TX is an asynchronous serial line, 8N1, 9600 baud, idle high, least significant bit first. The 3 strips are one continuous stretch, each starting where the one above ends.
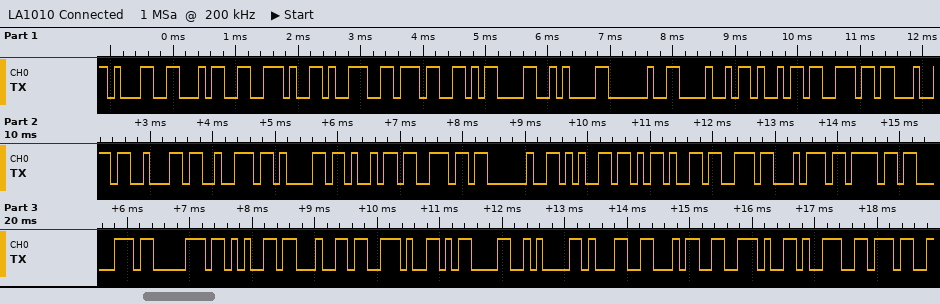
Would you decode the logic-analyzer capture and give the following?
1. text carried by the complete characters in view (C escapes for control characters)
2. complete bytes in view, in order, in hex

"14.97\r\n Hindbrain e-stopped.\r\n14.97"
31 34 2E 39 37 0D 0A 20 48 69 6E 64 62 72 61 69 6E 20 65 2D 73 74 6F 70 70 65 64 2E 0D 0A 31 34 2E 39 37
